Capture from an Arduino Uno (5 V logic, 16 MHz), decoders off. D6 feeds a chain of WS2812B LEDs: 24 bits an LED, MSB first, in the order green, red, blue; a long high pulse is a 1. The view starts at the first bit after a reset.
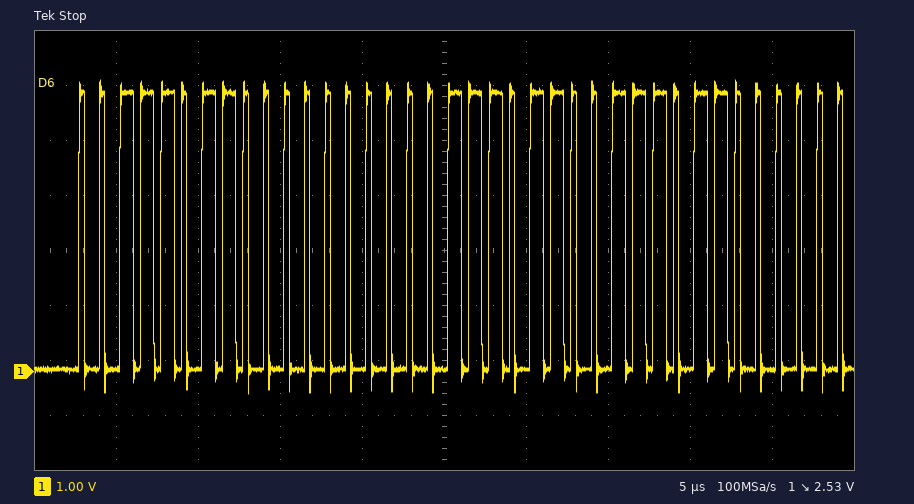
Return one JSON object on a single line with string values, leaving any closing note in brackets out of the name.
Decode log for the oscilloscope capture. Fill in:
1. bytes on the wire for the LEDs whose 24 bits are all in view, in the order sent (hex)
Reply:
{"bytes on the wire for the LEDs whose 24 bits are all in view, in the order sent": "3B 00 3B"}
